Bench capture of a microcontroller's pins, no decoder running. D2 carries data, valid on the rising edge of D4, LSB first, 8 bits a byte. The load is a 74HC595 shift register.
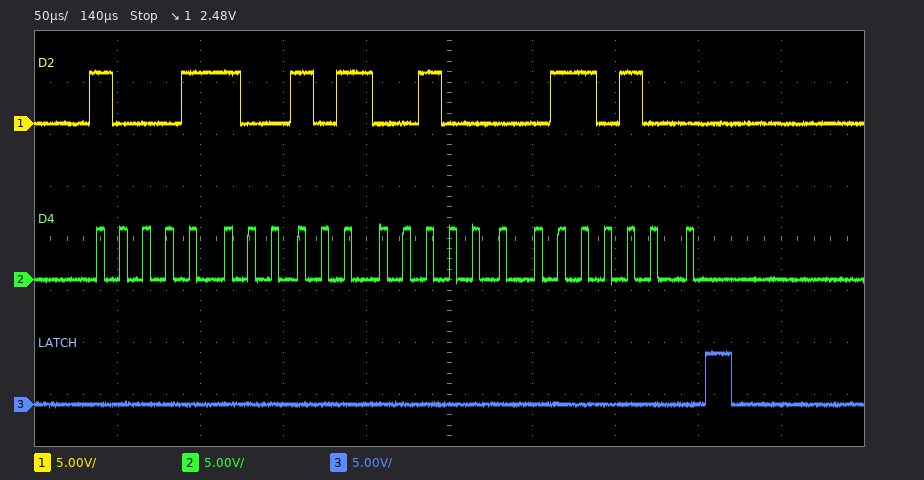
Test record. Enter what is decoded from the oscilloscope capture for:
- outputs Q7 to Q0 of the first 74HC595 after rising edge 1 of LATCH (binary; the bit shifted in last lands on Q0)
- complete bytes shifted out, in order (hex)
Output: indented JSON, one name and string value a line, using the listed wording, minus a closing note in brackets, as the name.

{
  "outputs Q7 to Q0 of the first 74HC595 after rising edge 1 of LATCH": "00110100",
  "complete bytes shifted out, in order": "0x31 0x25 0x2C"
}
